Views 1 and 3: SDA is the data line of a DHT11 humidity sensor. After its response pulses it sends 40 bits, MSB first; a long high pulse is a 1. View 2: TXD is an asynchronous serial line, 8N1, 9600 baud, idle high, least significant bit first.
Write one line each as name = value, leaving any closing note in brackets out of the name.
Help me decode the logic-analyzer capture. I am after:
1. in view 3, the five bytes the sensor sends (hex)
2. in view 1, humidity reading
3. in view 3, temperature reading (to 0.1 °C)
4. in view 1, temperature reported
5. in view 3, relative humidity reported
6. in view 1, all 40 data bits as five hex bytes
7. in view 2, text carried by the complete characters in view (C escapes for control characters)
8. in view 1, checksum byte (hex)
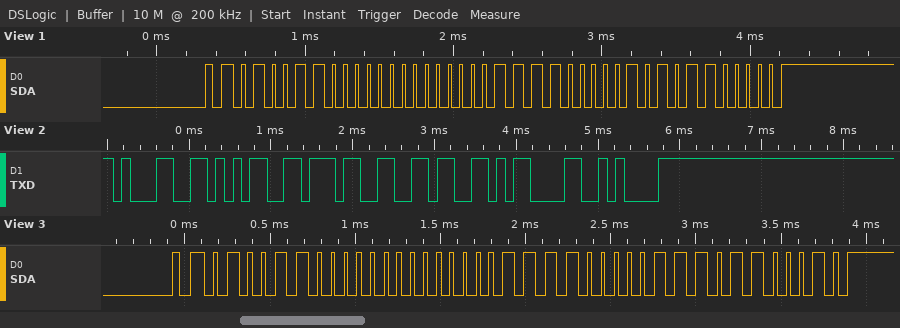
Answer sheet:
in view 3, the five bytes the sensor sends = 4C 00 0F 07 62
in view 1, humidity reading = 76 %
in view 3, temperature reading = 15.7 °C
in view 1, temperature reported = 15.5 °C
in view 3, relative humidity reported = 76 %
in view 1, all 40 data bits as five hex bytes = 4C 00 0F 05 60
in view 2, text carried by the complete characters in view = "1576\r\n"
in view 1, checksum byte = 0x60
